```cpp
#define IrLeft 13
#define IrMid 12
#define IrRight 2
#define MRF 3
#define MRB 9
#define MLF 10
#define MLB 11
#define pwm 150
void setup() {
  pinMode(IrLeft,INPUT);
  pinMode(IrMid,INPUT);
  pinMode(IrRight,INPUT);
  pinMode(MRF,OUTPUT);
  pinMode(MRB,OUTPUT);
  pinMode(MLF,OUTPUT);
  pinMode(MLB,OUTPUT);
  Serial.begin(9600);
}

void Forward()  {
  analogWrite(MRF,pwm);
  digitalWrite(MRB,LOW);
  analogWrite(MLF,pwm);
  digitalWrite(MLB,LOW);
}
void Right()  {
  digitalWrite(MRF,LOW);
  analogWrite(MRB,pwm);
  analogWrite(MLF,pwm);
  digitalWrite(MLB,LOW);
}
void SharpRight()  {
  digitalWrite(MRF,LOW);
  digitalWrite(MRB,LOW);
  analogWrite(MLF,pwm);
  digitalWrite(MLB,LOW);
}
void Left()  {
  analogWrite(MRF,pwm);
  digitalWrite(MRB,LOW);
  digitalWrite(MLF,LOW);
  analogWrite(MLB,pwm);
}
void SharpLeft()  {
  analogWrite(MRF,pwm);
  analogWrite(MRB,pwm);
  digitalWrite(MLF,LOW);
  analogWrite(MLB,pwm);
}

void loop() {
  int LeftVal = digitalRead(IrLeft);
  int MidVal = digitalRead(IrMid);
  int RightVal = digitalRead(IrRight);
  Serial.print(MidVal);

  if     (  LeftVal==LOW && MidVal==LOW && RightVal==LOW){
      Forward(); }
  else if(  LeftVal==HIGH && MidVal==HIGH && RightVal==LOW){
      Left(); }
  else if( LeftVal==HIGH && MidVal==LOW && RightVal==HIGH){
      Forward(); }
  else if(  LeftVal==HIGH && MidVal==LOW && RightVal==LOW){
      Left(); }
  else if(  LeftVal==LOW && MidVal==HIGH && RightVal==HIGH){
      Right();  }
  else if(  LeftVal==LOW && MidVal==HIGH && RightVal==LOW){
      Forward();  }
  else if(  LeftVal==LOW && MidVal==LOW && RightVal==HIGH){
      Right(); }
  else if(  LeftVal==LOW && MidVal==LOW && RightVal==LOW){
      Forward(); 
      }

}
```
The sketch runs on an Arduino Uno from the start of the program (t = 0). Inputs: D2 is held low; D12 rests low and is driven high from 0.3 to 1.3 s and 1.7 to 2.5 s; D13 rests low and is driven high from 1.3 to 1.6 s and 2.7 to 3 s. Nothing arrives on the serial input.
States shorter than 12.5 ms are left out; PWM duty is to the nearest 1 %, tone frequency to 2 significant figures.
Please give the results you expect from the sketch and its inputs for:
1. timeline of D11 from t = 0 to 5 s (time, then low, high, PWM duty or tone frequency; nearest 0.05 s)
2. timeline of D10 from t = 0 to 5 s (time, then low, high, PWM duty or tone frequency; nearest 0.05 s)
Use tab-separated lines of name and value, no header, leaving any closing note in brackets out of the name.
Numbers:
timeline of D11 from t = 0 to 5 s	0 s low; 1.3 s PWM 59 %; 1.6 s low; 2.7 s PWM 59 %; 3 s low
timeline of D10 from t = 0 to 5 s	0 s PWM 59 %; 1.3 s low; 1.6 s PWM 59 %; 2.7 s low; 3 s PWM 59 %
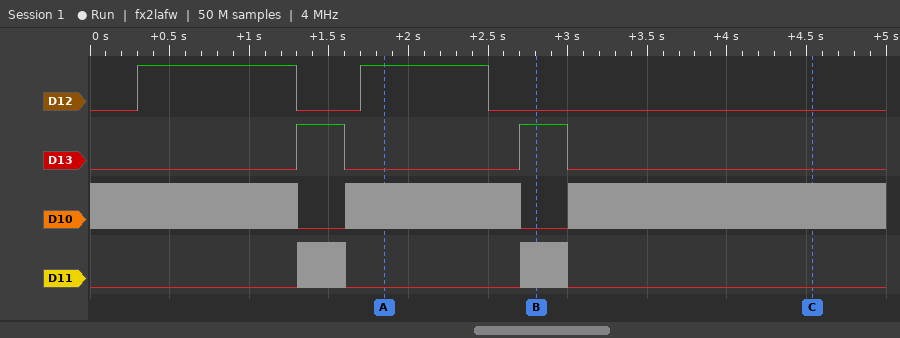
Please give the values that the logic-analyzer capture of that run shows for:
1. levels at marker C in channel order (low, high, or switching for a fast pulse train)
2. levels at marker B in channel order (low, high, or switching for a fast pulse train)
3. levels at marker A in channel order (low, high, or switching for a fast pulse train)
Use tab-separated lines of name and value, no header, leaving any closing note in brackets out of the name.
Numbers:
levels at marker C in channel order	D12 low, D13 low, D10 switching, D11 low
levels at marker B in channel order	D12 low, D13 high, D10 low, D11 switching
levels at marker A in channel order	D12 high, D13 low, D10 switching, D11 low
